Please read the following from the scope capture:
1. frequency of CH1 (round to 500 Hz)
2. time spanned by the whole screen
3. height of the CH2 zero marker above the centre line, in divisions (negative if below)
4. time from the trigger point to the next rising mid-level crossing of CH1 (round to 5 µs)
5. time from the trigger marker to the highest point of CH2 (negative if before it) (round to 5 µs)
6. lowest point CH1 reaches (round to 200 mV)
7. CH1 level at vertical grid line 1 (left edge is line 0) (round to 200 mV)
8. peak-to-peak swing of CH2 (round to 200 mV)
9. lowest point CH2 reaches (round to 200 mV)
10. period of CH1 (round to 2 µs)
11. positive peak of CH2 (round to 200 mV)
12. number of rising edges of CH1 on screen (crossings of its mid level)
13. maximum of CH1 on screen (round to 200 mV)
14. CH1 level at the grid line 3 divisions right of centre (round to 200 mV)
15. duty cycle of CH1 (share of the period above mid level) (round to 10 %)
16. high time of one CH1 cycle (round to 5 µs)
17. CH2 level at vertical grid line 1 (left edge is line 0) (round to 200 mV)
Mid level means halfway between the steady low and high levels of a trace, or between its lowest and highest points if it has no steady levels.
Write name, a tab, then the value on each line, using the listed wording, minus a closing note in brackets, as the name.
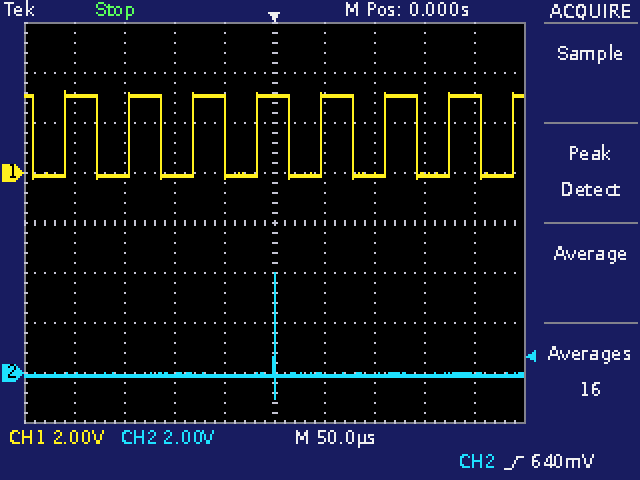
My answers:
frequency of CH1	15.5 kHz
time spanned by the whole screen	500 µs
height of the CH2 zero marker above the centre line, in divisions	-3.0 div
time from the trigger point to the next rising mid-level crossing of CH1	45 µs
time from the trigger marker to the highest point of CH2 (negative if before it)	0 µs
lowest point CH1 reaches	-200 mV
CH1 level at vertical grid line 1 (left edge is line 0)	3.0 V
peak-to-peak swing of CH2	5.0 V
lowest point CH2 reaches	-1.0 V
period of CH1	64 µs
positive peak of CH2	4.0 V
number of rising edges of CH1 on screen	8
maximum of CH1 on screen	3.2 V
CH1 level at the grid line 3 divisions right of centre	0.0 V
duty cycle of CH1 (share of the period above mid level)	50 %
high time of one CH1 cycle	30 µs
CH2 level at vertical grid line 1 (left edge is line 0)	0.0 V
